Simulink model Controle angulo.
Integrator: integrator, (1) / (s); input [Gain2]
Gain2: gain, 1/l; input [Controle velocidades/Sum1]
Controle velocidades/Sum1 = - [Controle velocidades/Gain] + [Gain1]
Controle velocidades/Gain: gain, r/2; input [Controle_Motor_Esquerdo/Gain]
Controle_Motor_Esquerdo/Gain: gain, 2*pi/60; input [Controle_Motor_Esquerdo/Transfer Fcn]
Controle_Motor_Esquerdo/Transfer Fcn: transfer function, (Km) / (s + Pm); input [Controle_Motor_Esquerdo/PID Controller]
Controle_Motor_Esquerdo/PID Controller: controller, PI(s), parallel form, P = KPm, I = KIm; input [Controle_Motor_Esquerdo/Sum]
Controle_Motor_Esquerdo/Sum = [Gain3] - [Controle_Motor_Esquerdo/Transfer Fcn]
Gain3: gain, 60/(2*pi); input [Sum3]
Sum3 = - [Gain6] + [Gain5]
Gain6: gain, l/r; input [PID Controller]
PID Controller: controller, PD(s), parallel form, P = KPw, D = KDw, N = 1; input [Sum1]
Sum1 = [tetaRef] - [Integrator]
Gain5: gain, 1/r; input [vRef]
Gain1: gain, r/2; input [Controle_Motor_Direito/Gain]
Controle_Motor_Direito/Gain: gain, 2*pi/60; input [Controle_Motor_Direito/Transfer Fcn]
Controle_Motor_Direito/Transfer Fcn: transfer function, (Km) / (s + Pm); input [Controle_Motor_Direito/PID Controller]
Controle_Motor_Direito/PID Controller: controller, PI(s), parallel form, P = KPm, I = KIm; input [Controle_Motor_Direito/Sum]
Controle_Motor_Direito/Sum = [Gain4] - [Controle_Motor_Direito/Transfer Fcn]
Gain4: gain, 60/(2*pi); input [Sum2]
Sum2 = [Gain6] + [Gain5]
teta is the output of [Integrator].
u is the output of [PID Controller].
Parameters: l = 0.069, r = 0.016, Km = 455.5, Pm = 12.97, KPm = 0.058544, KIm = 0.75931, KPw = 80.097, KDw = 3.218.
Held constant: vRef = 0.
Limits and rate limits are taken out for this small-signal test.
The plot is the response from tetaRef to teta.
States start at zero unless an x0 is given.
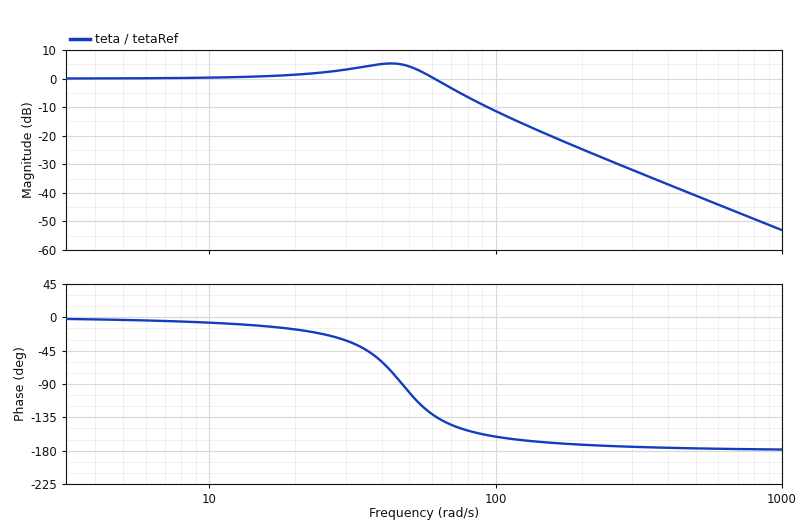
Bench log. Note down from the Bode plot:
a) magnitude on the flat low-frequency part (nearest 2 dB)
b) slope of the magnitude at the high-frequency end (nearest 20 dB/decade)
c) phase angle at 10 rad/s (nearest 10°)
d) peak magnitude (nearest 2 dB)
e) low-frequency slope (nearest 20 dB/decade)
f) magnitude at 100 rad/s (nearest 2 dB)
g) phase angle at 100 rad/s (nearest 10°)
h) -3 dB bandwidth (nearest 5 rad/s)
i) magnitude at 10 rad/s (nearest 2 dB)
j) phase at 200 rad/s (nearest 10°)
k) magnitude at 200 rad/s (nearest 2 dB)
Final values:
0 dB
-40 dB/decade
-10°
6 dB
0 dB/decade
-12 dB
-160°
70 rad/s
0 dB
-170°
-24 dB
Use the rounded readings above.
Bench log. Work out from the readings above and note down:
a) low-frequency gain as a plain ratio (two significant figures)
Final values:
1.0
